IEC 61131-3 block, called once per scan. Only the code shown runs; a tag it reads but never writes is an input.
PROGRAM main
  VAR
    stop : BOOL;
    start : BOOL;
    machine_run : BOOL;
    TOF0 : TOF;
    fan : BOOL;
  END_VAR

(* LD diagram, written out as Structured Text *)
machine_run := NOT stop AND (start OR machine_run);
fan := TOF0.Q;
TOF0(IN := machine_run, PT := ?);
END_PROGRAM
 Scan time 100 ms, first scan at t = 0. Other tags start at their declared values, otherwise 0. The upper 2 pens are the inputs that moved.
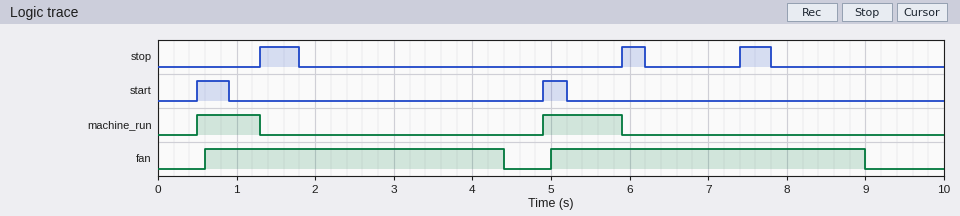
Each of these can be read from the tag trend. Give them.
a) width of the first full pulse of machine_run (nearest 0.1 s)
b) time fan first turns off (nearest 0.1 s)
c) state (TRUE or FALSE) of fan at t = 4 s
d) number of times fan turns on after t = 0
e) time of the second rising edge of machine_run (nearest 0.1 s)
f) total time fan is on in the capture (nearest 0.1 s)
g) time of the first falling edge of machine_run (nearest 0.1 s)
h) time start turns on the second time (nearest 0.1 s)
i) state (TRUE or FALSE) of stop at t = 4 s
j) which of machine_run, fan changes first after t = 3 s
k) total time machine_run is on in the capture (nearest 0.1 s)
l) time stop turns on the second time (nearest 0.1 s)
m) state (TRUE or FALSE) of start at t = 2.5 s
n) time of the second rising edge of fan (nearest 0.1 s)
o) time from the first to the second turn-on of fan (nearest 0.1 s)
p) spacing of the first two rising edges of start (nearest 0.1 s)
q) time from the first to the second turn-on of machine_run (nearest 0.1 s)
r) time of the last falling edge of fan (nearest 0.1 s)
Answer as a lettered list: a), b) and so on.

a) 0.8 s
b) 4.4 s
c) TRUE
d) 2
e) 4.9 s
f) 7.8 s
g) 1.3 s
h) 4.9 s
i) FALSE
j) fan
k) 1.8 s
l) 5.9 s
m) FALSE
n) 5.0 s
o) 4.4 s
p) 4.4 s
q) 4.4 s
r) 9.0 s
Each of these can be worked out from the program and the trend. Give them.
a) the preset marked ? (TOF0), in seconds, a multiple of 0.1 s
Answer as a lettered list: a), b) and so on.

a) 3.0 s
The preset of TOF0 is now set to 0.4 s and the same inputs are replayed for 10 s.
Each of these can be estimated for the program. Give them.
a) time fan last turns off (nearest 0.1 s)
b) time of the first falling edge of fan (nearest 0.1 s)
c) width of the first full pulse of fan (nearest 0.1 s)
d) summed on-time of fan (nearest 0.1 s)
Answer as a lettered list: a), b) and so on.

a) 6.4 s
b) 1.8 s
c) 1.2 s
d) 2.6 s
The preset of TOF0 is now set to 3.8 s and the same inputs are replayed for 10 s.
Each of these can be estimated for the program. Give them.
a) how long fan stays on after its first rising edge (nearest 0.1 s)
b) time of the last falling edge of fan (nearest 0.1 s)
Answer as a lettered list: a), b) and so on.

a) 9.2 s
b) 9.8 s
